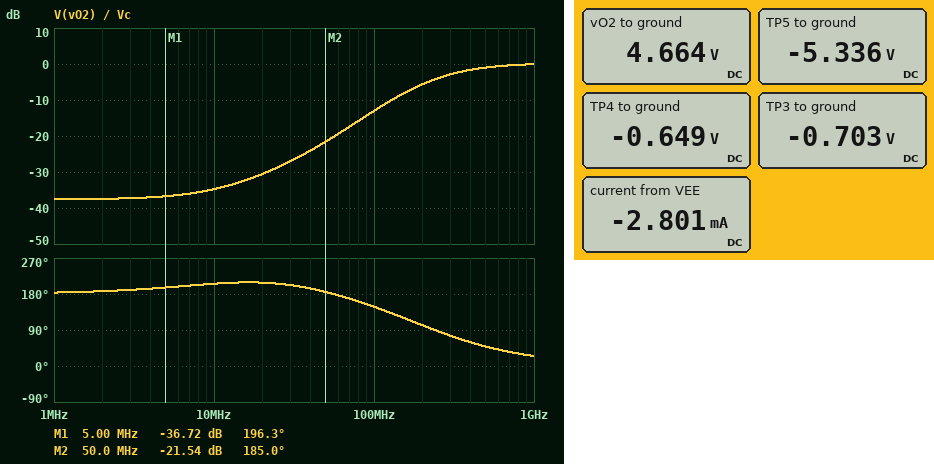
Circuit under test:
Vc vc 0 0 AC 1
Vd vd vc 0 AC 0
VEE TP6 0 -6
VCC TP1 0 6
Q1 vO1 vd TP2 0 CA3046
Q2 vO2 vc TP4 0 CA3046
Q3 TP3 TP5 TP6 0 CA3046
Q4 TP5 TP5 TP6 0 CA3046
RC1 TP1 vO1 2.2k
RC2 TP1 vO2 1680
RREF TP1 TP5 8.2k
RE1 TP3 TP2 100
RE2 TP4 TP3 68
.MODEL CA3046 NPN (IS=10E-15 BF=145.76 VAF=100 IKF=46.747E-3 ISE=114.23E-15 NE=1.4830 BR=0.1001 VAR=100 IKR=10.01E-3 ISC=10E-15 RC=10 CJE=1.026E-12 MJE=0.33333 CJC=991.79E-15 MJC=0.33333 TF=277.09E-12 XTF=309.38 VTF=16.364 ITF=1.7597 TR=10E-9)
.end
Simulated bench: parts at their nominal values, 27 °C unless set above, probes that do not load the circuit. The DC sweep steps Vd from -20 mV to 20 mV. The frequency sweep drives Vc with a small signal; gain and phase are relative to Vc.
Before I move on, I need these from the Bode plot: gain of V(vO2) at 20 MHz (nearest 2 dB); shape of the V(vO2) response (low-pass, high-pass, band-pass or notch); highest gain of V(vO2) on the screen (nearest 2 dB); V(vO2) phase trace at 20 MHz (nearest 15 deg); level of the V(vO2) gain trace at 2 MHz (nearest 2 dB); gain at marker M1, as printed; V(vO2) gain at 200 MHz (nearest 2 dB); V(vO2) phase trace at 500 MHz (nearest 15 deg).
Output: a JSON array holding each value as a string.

["-30 dB", "high-pass", "0 dB", "210 deg", "-38 dB", "-36.72 dB", "-6 dB", "45 deg"]
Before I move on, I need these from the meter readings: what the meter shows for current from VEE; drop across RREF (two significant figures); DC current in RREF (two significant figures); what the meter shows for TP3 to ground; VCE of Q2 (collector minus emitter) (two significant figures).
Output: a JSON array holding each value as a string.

["-2.801 mA", "11 V", "1.4 mA", "-0.703 V", "5.3 V"]
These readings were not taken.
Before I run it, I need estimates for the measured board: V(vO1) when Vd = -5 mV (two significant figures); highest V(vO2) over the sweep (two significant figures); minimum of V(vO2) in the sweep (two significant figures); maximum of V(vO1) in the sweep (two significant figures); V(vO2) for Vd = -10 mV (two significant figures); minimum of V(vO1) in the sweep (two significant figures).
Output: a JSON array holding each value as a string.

["4.7 V", "4.8 V", "4.5 V", "4.8 V", "4.6 V", "4.5 V"]
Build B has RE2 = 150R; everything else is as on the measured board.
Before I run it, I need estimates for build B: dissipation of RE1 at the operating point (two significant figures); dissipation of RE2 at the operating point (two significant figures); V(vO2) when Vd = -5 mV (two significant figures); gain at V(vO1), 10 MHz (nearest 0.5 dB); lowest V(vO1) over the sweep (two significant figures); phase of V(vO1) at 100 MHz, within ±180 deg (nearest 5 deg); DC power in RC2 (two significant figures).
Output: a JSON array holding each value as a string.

["67 µW", "54 µW", "5.0 V", "-32.5 dB", "4.1 V", "140 deg", "590 µW"]
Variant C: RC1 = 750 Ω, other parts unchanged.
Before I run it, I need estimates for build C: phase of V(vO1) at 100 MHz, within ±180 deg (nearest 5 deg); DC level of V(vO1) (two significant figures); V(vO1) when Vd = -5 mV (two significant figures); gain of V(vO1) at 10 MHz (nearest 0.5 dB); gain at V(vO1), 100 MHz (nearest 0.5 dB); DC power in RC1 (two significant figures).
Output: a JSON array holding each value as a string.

["130 deg", "5.5 V", "5.6 V", "-44.5 dB", "-20.0 dB", "280 µW"]
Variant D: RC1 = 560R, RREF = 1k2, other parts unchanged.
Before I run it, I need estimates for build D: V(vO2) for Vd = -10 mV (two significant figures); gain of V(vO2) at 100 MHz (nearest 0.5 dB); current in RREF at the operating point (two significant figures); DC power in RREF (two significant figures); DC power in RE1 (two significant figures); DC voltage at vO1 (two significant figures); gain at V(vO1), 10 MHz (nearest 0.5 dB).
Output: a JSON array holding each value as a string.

["-570 mV", "0 dB", "9.4 mA", "110 mW", "1.6 mW", "3.8 V", "-33.0 dB"]
